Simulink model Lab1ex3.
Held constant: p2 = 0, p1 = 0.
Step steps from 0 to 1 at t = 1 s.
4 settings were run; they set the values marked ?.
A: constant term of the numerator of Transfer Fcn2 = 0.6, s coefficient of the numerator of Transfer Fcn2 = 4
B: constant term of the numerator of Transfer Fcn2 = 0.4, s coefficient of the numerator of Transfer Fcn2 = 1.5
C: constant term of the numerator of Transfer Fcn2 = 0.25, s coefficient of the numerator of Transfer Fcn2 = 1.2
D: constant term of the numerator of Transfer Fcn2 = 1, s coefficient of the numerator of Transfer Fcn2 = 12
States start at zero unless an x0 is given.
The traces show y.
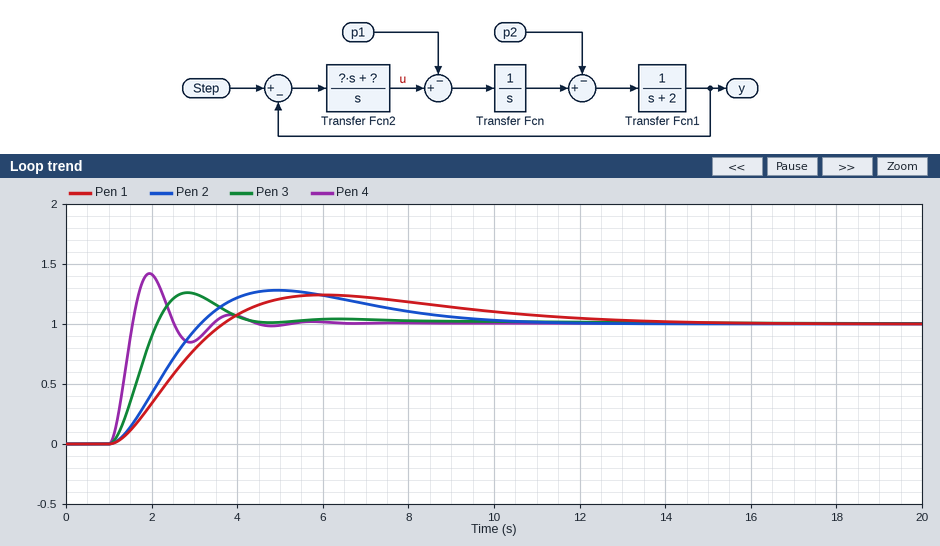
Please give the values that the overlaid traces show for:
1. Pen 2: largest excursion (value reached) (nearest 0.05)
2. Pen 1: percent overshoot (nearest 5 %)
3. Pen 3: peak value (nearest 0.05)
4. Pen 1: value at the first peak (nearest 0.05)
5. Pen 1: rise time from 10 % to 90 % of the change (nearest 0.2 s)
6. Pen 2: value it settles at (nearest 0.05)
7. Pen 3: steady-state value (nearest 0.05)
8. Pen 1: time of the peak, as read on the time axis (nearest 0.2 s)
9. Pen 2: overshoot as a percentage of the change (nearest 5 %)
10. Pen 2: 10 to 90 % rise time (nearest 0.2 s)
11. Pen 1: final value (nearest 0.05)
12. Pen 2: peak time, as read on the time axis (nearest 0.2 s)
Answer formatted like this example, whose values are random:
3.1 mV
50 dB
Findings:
1.30
25 %
1.25
1.25
1.8 s
1.00
1.00
6.0 s
30 %
1.4 s
1.00
5.0 s
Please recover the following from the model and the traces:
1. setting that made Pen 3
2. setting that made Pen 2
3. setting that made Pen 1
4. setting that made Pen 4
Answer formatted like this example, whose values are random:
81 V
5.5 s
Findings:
A
B
C
D
